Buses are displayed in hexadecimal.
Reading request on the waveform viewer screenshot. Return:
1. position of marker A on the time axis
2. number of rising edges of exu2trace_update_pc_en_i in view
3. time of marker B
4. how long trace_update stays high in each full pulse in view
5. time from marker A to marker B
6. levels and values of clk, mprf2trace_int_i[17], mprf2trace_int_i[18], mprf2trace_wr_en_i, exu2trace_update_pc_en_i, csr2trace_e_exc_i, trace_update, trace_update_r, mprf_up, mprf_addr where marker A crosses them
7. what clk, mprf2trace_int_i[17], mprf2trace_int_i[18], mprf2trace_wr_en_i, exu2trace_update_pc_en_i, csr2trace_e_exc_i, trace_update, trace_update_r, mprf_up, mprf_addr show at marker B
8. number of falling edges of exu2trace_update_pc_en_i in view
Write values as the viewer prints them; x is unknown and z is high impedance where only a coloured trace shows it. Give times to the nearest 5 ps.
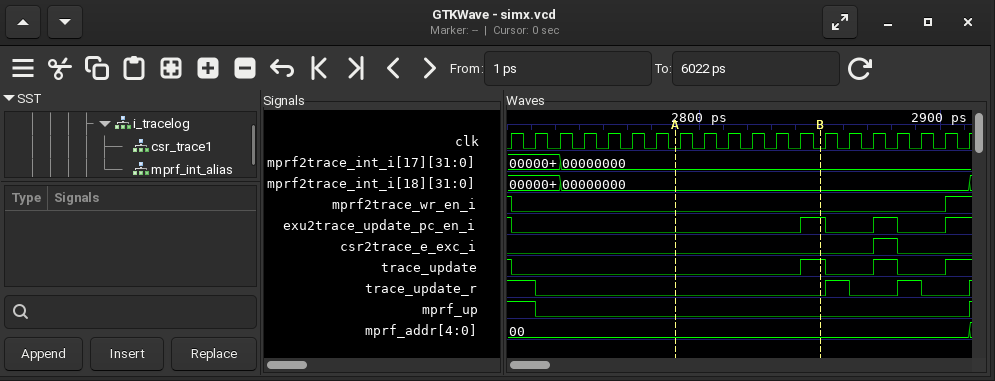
2790 ps
3
2850 ps
10 ps, 10 ps
60 ps
clk=0, mprf2trace_int_i[17]=00000000, mprf2trace_int_i[18]=00000000, mprf2trace_wr_en_i=0, exu2trace_update_pc_en_i=0, csr2trace_e_exc_i=0, trace_update=0, trace_update_r=0, mprf_up=0, mprf_addr=00
clk=0, mprf2trace_int_i[17]=00000000, mprf2trace_int_i[18]=00000000, mprf2trace_wr_en_i=0, exu2trace_update_pc_en_i=1, csr2trace_e_exc_i=0, trace_update=1, trace_update_r=0, mprf_up=0, mprf_addr=00
3
